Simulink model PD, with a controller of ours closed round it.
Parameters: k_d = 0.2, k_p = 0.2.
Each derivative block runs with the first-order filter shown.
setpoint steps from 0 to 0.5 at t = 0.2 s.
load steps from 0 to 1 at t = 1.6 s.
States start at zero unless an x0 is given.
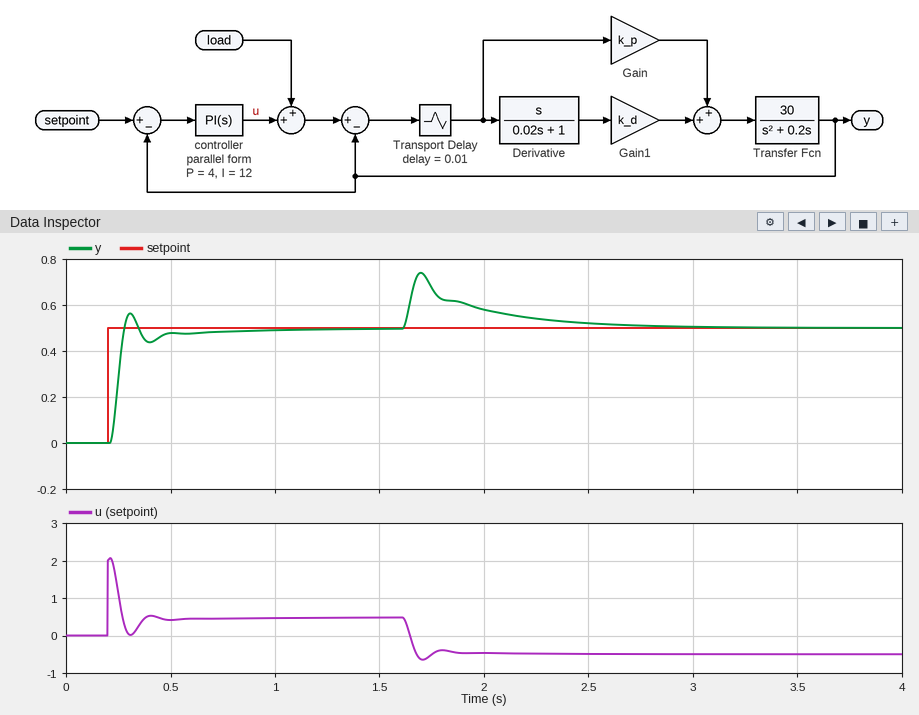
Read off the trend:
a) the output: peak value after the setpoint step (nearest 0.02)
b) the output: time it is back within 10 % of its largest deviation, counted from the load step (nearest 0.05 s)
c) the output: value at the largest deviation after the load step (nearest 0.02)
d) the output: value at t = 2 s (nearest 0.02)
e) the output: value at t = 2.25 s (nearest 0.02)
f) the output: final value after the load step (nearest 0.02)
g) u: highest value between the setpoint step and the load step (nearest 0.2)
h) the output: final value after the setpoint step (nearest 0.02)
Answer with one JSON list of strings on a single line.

["0.56", "0.85 s", "0.74", "0.58", "0.54", "0.50", "2.0", "0.50"]
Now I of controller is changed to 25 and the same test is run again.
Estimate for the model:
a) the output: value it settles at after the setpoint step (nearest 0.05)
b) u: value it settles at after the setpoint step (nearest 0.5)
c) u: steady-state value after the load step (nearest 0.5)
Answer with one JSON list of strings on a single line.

["0.50", "0.5", "-0.5"]
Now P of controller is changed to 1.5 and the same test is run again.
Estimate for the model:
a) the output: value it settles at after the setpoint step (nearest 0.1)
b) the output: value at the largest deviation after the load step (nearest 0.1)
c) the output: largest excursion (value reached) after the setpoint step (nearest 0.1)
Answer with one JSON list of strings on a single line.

["0.5", "0.9", "0.5"]
